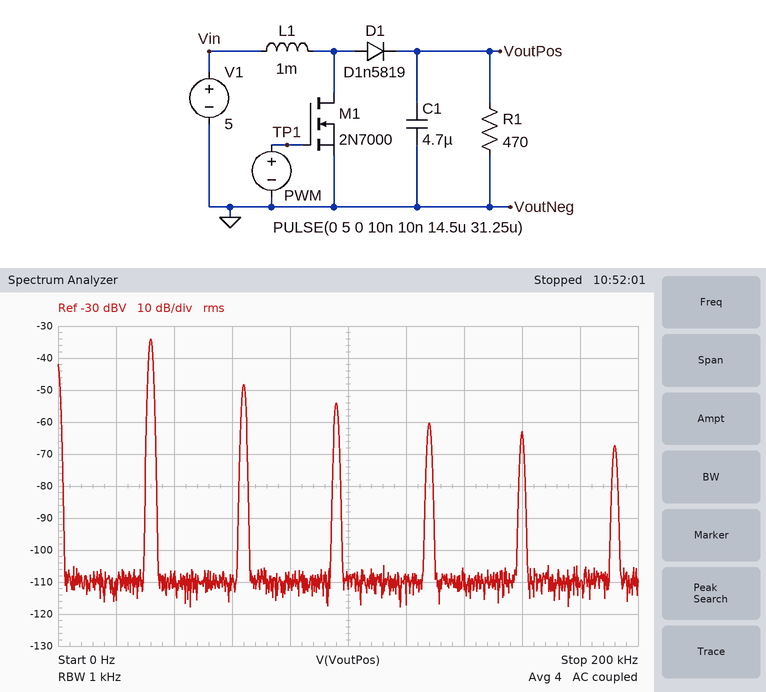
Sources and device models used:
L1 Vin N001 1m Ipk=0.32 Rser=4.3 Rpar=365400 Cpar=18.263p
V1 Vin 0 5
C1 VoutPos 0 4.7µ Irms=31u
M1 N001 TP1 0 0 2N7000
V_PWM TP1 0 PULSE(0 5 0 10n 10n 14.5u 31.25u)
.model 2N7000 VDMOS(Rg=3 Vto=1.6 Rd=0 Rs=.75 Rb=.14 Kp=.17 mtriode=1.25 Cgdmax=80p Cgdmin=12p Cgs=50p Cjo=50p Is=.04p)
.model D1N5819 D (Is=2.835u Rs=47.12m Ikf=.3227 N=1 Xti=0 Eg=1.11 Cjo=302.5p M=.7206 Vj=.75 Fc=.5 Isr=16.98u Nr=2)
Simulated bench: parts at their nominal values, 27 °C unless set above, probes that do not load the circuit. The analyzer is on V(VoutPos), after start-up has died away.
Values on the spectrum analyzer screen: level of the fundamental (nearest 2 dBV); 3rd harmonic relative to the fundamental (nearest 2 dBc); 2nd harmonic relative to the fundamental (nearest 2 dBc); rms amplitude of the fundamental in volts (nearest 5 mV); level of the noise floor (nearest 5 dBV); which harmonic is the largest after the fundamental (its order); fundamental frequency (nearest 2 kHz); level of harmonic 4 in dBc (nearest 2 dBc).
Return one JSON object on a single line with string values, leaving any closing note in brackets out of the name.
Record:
{"level of the fundamental": "-34 dBV", "3rd harmonic relative to the fundamental": "-20 dBc", "2nd harmonic relative to the fundamental": "-14 dBc", "rms amplitude of the fundamental in volts": "20 mV", "level of the noise floor": "-110 dBV", "which harmonic is the largest after the fundamental": "2", "fundamental frequency": "32 kHz", "level of harmonic 4 in dBc": "-26 dBc"}
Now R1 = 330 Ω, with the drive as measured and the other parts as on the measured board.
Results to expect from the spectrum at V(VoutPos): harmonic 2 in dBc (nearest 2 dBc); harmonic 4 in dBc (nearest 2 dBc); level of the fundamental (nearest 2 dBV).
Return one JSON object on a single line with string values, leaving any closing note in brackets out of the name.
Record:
{"harmonic 2 in dBc": "-16 dBc", "harmonic 4 in dBc": "-28 dBc", "level of the fundamental": "-32 dBV"}
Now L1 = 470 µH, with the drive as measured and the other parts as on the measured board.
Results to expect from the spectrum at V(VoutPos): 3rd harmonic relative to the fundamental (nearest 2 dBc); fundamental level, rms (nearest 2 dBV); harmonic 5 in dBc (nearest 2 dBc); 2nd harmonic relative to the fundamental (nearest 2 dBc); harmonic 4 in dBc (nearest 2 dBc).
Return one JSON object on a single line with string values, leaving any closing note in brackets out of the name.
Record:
{"3rd harmonic relative to the fundamental": "-18 dBc", "fundamental level, rms": "-30 dBV", "harmonic 5 in dBc": "-26 dBc", "2nd harmonic relative to the fundamental": "-10 dBc", "harmonic 4 in dBc": "-24 dBc"}
